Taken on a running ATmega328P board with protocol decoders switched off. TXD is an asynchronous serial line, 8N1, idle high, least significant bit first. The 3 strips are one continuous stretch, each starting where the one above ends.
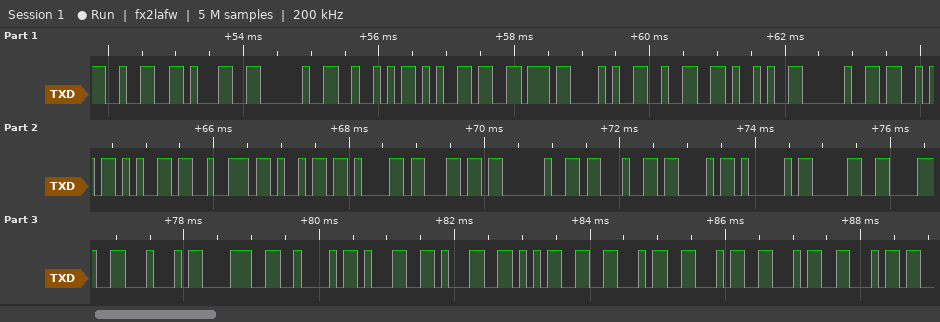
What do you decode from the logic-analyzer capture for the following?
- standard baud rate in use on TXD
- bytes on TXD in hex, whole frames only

9600 baud
32 31 20 52 65 76 28 32 29 20 53 65 72 69 61 6C 20 23 43 41 30 38 44 38 42 31 31 35 46 46 46 46
